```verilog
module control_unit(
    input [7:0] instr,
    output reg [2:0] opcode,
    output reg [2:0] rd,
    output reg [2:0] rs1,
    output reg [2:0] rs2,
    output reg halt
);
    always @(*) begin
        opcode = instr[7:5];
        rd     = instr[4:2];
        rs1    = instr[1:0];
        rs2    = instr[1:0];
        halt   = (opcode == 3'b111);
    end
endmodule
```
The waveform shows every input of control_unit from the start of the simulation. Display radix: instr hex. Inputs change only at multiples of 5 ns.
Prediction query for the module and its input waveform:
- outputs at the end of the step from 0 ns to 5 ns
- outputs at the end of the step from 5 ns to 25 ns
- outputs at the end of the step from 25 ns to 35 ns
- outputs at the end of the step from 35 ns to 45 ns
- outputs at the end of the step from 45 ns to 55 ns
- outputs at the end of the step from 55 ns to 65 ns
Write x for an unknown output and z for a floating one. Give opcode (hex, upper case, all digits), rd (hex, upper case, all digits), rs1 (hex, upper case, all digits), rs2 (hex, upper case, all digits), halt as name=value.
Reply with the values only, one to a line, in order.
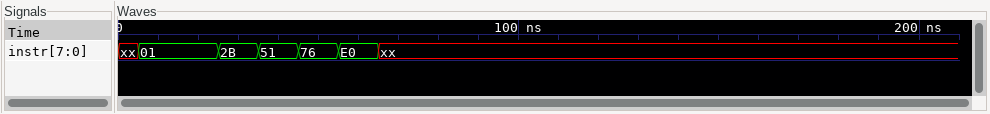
opcode=x, rd=x, rs1=x, rs2=x, halt=x
opcode=0, rd=0, rs1=1, rs2=1, halt=0
opcode=1, rd=2, rs1=3, rs2=3, halt=0
opcode=2, rd=4, rs1=1, rs2=1, halt=0
opcode=3, rd=5, rs1=2, rs2=2, halt=0
opcode=7, rd=0, rs1=0, rs2=0, halt=1
